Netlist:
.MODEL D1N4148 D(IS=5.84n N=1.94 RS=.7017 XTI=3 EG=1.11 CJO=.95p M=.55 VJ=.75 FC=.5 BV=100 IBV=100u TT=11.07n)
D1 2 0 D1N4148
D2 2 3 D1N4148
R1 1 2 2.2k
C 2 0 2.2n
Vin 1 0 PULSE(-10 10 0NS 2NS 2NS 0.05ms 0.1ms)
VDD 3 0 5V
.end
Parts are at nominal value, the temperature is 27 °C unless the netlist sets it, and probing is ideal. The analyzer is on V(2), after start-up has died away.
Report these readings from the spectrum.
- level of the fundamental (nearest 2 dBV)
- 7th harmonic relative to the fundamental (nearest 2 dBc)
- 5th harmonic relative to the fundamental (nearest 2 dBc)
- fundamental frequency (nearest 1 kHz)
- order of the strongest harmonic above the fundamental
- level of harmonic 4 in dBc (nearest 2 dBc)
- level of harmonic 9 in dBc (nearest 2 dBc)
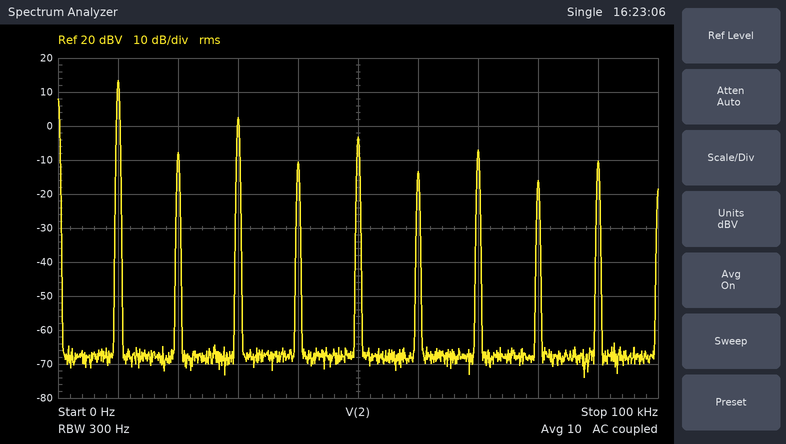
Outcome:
14 dBV
-20 dBc
-16 dBc
10 kHz
3
-24 dBc
-24 dBc
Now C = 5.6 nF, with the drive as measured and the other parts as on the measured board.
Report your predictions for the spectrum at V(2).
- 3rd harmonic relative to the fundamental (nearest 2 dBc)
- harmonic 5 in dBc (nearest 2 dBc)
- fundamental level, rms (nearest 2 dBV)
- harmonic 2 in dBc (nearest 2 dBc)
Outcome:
-12 dBc
-20 dBc
12 dBV
-16 dBc
